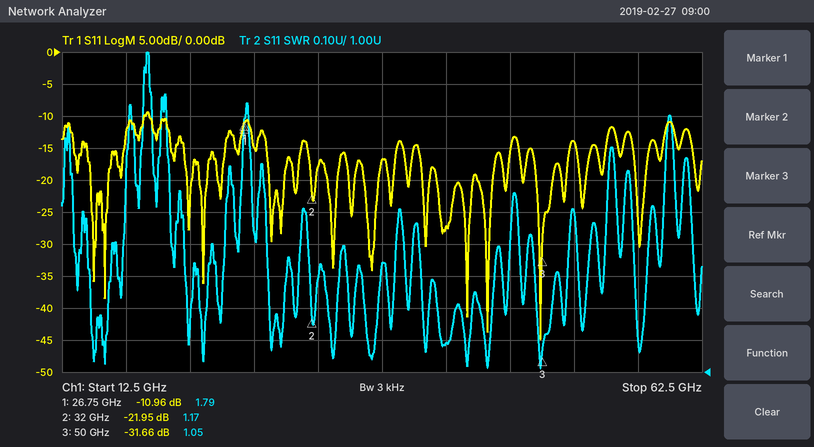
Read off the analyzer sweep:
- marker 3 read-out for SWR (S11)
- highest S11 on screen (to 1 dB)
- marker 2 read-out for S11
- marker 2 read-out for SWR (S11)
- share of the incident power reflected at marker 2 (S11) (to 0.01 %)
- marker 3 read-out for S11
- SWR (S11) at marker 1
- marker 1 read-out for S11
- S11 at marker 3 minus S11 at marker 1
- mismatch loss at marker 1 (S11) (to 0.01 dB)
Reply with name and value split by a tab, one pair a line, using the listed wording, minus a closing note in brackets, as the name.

marker 3 read-out for SWR	1.05
highest S11 on screen	-9 dB
marker 2 read-out for S11	-21.95 dB
marker 2 read-out for SWR	1.17
share of the incident power reflected at marker 2 (S11)	0.64 %
marker 3 read-out for S11	-31.66 dB
SWR (S11) at marker 1	1.79
marker 1 read-out for S11	-10.96 dB
S11 at marker 3 minus S11 at marker 1	-20.70 dB
mismatch loss at marker 1 (S11)	0.36 dB
